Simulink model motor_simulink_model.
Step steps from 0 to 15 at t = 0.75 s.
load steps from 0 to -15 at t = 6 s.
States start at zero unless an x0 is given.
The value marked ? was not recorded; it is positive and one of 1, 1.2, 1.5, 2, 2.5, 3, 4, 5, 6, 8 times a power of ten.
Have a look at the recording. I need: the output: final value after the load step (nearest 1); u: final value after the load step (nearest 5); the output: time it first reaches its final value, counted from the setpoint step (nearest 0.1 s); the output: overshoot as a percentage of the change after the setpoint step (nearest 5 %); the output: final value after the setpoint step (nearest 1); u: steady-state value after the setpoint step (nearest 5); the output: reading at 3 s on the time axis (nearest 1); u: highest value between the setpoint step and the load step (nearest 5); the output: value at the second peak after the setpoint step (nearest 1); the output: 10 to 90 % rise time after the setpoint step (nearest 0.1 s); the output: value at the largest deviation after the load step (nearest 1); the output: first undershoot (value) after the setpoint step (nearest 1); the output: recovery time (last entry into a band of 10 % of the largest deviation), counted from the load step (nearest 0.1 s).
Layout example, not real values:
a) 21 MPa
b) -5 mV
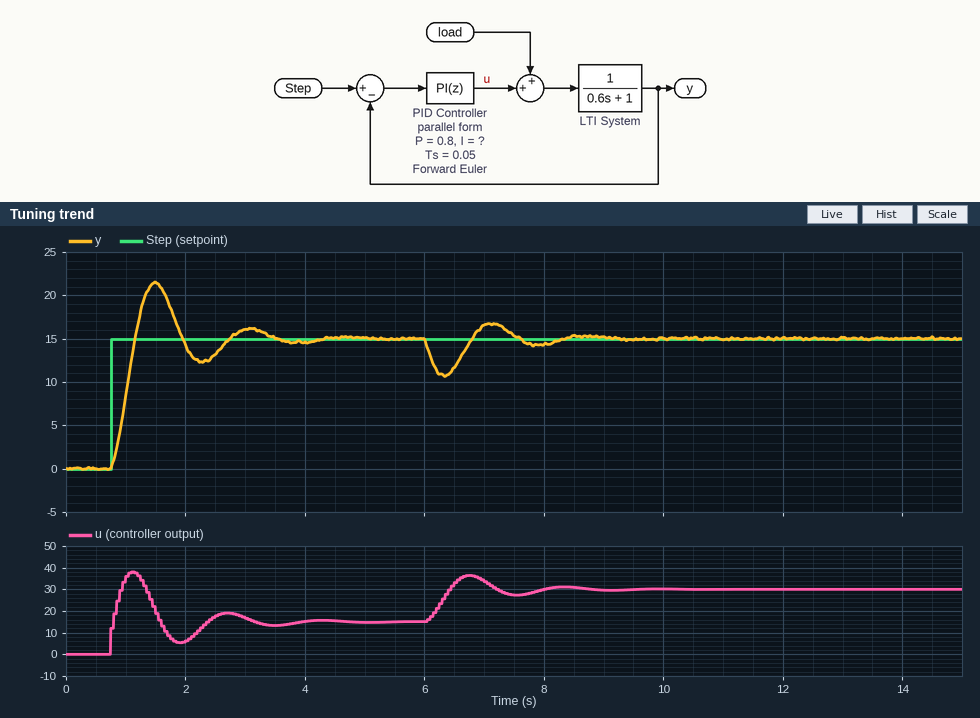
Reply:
a) 15
b) 30
c) 0.4 s
d) 45 %
e) 15
f) 15
g) 16
h) 40
i) 16
j) 0.3 s
k) 11
l) 12
m) 2.2 s
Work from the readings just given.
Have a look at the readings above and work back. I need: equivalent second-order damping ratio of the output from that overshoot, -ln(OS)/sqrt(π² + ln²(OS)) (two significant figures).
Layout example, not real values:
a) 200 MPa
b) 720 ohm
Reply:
a) 0.25
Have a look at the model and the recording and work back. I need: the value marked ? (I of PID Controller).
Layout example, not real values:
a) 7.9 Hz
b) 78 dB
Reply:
a) 10
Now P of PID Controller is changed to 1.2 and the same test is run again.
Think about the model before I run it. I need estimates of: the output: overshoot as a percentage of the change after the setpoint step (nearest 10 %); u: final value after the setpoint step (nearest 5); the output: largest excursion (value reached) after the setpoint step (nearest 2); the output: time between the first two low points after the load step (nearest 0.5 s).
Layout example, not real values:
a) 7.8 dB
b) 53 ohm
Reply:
a) 30 %
b) 15
c) 20
d) 1.5 s
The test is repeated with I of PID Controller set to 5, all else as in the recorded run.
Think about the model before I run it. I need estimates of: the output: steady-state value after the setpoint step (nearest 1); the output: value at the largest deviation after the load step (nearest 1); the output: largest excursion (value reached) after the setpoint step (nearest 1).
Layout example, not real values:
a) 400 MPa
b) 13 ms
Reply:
a) 15
b) 10
c) 18
